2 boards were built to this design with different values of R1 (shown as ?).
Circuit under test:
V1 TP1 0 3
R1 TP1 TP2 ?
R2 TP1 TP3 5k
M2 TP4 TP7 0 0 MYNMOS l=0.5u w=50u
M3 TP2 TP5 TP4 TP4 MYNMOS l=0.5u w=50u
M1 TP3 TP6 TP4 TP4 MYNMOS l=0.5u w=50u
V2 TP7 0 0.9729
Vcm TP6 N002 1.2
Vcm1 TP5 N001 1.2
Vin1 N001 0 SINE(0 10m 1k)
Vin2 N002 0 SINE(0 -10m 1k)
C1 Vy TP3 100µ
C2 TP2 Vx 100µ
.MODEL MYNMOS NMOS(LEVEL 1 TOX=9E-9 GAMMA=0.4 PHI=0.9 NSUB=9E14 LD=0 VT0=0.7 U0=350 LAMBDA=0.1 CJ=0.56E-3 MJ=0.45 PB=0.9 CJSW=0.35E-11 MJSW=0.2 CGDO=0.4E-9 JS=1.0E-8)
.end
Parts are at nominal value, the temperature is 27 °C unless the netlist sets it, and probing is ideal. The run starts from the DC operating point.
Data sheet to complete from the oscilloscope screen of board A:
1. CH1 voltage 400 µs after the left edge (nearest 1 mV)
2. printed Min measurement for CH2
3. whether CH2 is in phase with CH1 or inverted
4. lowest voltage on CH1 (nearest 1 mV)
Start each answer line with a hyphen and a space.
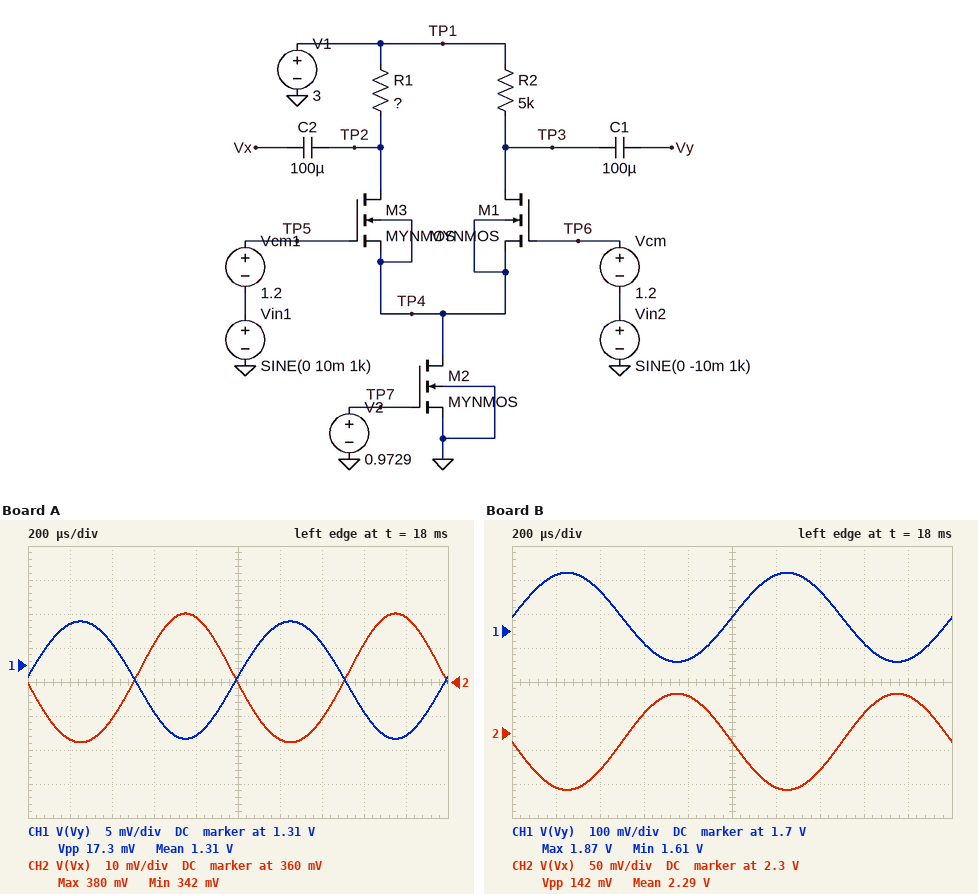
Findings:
- 1.313 V
- 342 mV
- inverted
- 1.299 V
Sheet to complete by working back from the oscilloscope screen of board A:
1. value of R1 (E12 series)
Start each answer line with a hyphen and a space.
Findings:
- 15 kΩ
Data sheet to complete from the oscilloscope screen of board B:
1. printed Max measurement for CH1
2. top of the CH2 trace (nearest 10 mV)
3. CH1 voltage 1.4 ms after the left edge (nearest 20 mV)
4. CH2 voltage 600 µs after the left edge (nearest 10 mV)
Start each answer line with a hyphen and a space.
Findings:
- 1.87 V
- 2.36 V
- 1.82 V
- 2.33 V
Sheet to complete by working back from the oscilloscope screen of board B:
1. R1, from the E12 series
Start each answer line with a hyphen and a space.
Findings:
- 2.7 kΩ
